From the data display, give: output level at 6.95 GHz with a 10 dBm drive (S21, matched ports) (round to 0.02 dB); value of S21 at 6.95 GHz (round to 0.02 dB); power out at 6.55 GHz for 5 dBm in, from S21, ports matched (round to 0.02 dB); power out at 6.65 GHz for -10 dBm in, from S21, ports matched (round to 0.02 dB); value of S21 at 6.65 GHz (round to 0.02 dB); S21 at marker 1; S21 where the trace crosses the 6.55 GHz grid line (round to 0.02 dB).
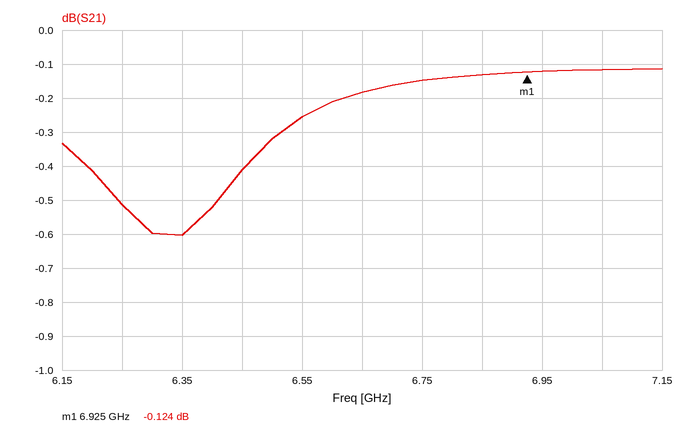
9.88 dBm
-0.12 dB
4.74 dBm
-10.18 dBm
-0.18 dB
-0.124 dB
-0.26 dB
